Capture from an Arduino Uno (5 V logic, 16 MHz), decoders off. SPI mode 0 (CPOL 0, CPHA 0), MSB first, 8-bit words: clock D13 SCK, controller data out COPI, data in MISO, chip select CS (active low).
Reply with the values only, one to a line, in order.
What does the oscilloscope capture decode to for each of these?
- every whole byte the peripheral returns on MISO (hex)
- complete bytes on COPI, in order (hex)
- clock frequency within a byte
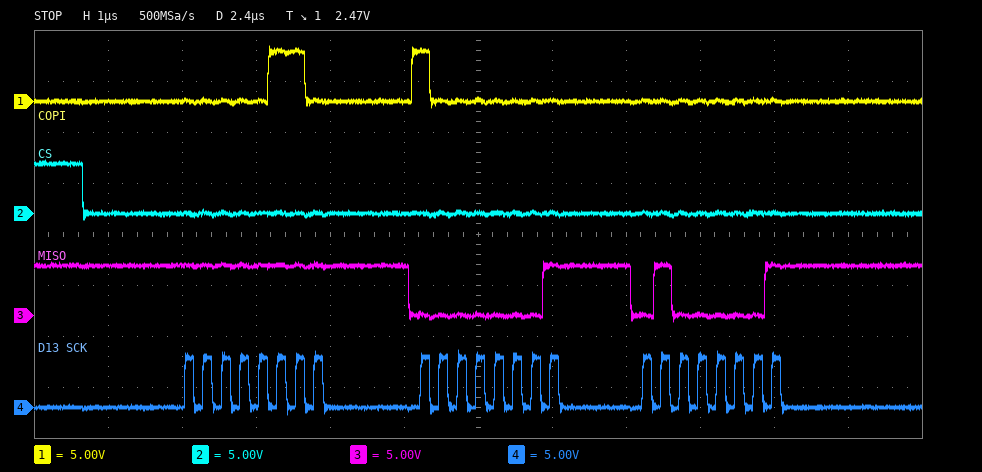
FF 01 41
06 80 00
4 MHz
